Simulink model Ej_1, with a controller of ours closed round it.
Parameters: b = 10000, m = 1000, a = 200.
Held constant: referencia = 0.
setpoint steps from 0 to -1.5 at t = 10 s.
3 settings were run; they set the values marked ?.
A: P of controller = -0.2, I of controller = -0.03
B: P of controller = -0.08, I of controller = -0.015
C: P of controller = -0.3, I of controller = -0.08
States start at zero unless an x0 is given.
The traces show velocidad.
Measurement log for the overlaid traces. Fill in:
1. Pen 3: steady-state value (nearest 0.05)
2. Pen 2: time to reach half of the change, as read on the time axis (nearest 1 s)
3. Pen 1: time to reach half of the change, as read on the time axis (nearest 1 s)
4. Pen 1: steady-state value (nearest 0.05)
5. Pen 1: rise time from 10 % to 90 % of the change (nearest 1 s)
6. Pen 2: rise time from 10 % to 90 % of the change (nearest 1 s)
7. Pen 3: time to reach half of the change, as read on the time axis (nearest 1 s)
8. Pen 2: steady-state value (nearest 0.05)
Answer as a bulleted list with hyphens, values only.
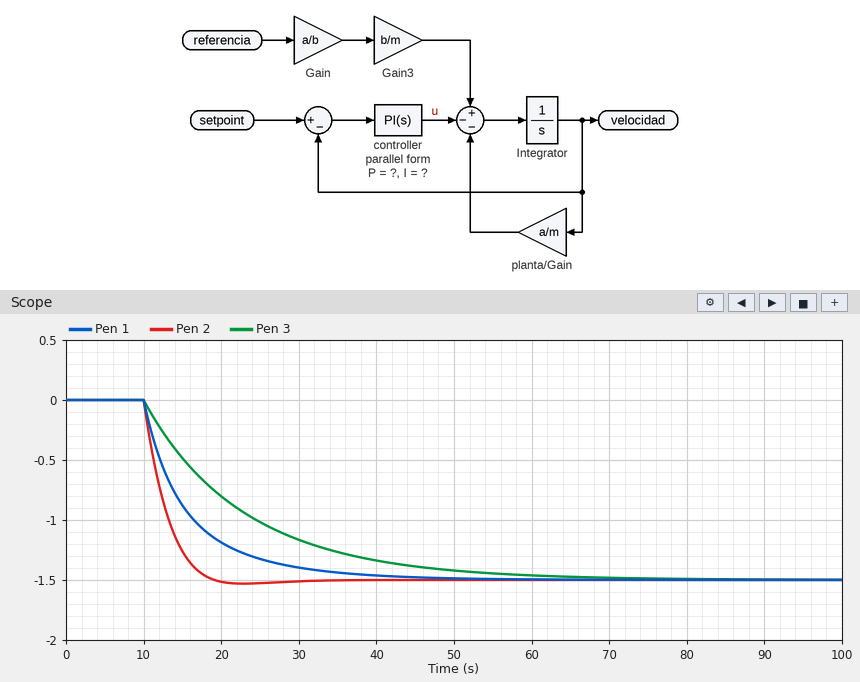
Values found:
- -1.50
- 12 s
- 14 s
- -1.50
- 16 s
- 6 s
- 19 s
- -1.50
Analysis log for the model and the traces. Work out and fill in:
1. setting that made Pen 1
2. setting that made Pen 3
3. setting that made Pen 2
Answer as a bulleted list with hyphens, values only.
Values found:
- A
- B
- C
